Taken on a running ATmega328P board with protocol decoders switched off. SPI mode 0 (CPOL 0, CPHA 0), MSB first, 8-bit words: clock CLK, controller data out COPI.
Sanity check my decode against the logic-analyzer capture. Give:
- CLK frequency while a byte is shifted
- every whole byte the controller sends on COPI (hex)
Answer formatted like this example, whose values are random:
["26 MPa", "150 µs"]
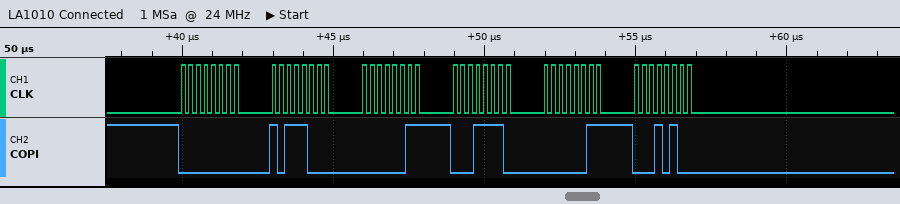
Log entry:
["4 MHz", "00 B8 03 1E 03 14"]
